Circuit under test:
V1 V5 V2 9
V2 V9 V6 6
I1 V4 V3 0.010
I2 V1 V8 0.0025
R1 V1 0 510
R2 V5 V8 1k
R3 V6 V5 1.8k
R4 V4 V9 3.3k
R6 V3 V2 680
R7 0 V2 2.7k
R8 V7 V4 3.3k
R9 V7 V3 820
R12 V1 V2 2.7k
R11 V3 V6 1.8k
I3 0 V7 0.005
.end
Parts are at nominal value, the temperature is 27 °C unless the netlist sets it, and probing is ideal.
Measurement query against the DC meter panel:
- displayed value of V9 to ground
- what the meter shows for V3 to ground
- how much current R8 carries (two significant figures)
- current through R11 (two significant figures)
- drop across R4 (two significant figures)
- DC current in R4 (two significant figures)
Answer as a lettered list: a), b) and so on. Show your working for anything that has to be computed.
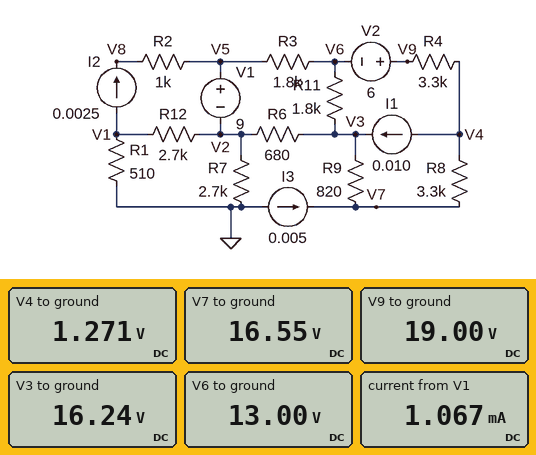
a) 19.00 V
b) 16.24 V
c) (16.55 V - 1.271 V) / 3.3 kΩ = 4.6 mA
d) (16.24 V - 13 V) / 1.8 kΩ = 1.8 mA
e) 19 V - 1.271 V = 18 V
f) (19 V - 1.271 V) / 3.3 kΩ = 5.4 mA
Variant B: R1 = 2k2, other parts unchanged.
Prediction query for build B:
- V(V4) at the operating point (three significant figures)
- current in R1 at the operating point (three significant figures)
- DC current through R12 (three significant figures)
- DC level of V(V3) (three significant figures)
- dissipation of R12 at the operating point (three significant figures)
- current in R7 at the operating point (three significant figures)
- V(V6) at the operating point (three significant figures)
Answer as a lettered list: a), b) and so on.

a) 1.96 V
b) 888 µA
c) 3.39 mA
d) 16.9 V
e) 31.0 mW
f) 4.11 mA
g) 13.7 V
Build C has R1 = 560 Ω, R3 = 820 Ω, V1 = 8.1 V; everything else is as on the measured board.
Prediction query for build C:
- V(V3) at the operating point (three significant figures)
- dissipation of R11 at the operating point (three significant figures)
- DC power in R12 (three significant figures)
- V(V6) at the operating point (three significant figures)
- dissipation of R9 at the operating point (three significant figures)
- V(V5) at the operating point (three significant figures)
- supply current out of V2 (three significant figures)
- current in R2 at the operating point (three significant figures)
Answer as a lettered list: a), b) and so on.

a) 16.9 V
b) 2.16 mW
c) 35.6 mW
d) 14.9 V
e) 242 µW
f) 18.5 V
g) 5.54 mA
h) 2.50 mA
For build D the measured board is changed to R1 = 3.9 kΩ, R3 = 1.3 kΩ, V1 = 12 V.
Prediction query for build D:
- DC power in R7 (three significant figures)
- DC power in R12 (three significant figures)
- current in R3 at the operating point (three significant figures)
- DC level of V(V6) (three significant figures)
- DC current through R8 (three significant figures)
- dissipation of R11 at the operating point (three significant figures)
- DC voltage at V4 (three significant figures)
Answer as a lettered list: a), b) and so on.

a) 49.3 mW
b) 28.1 mW
c) 4.96 mA
d) 17.1 V
e) 4.36 mA
f) 835 µW
g) 4.47 V
